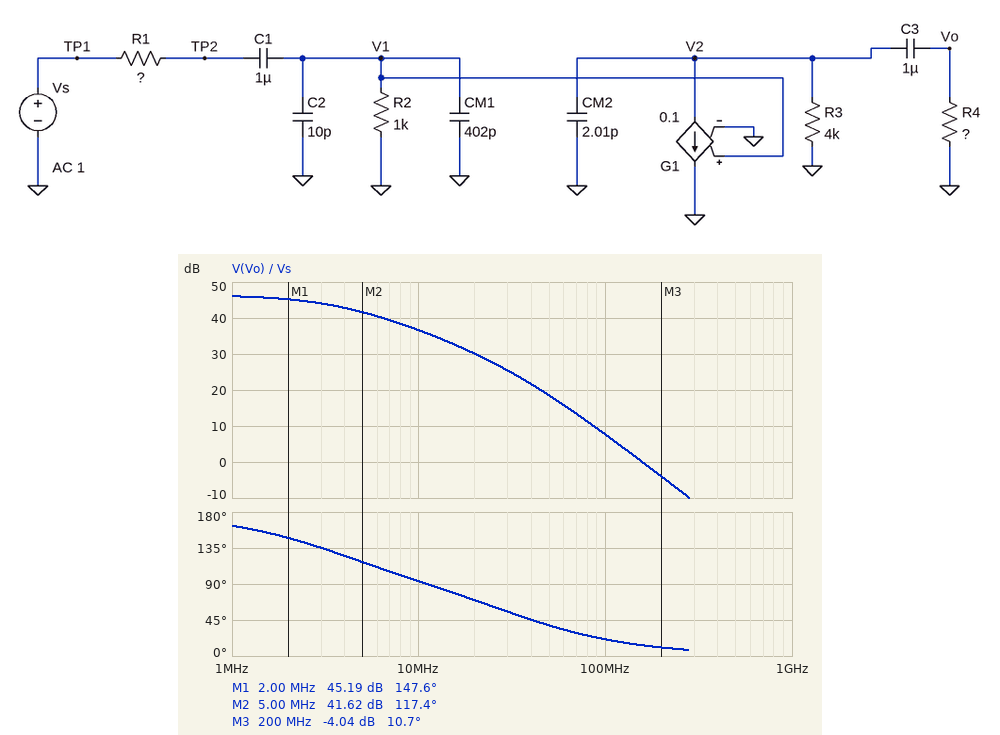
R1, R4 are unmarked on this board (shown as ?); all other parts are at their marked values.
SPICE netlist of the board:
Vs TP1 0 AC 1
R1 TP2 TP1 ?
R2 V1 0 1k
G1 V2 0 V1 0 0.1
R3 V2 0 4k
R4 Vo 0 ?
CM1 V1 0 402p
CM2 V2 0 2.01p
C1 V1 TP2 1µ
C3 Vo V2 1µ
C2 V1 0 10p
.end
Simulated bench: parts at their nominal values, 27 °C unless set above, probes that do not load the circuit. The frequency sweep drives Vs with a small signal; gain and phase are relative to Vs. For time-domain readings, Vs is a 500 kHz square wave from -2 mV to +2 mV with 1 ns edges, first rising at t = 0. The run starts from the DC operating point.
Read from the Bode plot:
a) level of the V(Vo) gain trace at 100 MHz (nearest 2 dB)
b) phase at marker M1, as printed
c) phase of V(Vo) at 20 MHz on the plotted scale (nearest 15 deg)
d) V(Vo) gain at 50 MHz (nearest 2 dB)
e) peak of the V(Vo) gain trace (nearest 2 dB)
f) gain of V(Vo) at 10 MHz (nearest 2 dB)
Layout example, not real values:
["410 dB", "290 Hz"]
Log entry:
["8 dB", "147.6 deg", "75 deg", "18 dB", "46 dB", "36 dB"]
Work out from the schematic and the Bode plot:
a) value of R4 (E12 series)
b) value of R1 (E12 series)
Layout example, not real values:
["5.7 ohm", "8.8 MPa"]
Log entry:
["5.6 kΩ", "120 Ω"]
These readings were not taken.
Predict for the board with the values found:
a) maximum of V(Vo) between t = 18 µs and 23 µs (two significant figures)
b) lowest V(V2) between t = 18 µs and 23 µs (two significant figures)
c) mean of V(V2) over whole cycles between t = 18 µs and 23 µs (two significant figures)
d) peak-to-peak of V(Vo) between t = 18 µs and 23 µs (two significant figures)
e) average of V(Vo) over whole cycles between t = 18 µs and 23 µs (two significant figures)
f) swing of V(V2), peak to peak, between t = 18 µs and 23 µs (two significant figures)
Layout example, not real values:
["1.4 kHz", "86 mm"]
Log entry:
["9.0 mV", "-830 mV", "-410 mV", "830 mV", "-410 mV", "830 mV"]
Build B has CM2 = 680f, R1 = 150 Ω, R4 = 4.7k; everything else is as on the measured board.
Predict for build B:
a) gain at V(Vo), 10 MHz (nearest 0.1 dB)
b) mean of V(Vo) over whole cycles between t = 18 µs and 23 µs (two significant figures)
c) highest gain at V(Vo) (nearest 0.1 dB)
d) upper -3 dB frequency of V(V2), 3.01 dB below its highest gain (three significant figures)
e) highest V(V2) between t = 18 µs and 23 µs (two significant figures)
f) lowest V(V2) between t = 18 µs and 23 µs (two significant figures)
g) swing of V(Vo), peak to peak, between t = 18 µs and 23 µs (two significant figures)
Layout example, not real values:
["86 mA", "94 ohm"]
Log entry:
["34.5 dB", "-370 mV", "45.5 dB", "2.96 MHz", "6.3 mV", "-750 mV", "750 mV"]
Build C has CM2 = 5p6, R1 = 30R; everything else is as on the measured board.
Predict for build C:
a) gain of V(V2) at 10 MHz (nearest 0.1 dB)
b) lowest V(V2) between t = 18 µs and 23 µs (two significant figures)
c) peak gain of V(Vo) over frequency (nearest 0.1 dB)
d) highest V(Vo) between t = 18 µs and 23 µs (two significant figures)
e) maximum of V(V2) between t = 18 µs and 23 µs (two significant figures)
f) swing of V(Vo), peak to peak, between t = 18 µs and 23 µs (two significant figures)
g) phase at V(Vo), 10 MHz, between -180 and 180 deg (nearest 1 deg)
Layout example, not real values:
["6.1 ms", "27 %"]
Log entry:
["42.9 dB", "-900 mV", "47.1 dB", "11 mV", "8.8 mV", "910 mV", "104 deg"]
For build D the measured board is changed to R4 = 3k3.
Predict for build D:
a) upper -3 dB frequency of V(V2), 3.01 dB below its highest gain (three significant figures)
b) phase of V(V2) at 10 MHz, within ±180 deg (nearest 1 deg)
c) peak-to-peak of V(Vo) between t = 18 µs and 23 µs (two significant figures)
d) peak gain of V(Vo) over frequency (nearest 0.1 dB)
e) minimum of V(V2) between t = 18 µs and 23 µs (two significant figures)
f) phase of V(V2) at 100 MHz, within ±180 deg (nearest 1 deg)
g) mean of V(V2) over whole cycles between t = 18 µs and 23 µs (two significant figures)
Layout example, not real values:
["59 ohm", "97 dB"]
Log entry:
["3.58 MHz", "97 deg", "650 mV", "44.2 dB", "-640 mV", "26 deg", "-320 mV"]
